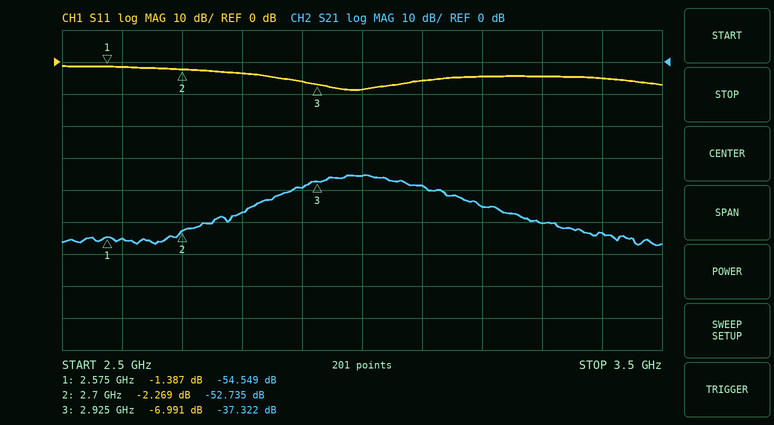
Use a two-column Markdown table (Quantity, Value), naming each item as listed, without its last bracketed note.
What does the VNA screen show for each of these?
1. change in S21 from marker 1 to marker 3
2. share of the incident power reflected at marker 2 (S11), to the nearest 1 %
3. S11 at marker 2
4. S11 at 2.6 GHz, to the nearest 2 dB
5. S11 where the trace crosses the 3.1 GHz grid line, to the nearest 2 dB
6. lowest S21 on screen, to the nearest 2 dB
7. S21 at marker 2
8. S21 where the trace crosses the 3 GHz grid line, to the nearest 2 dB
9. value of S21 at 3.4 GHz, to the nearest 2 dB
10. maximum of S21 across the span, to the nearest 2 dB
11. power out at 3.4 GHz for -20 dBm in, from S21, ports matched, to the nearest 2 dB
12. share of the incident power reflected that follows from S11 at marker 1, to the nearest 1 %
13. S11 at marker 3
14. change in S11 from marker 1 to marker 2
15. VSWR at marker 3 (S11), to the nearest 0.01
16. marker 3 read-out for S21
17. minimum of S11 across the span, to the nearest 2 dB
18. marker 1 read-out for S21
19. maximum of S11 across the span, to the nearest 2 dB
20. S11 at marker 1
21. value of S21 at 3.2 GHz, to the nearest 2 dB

| Quantity | Value |
|---|---|
| change in S21 from marker 1 to marker 3 | 17.227 dB |
| share of the incident power reflected at marker 2 (S11), to the nearest 1 % | 59 % |
| S11 at marker 2 | -2.269 dB |
| S11 at 2.6 GHz, to the nearest 2 dB | -2 dB |
| S11 where the trace crosses the 3.1 GHz grid line, to the nearest 2 dB | -6 dB |
| lowest S21 on screen, to the nearest 2 dB | -58 dB |
| S21 at marker 2 | -52.735 dB |
| S21 where the trace crosses the 3 GHz grid line, to the nearest 2 dB | -36 dB |
| value of S21 at 3.4 GHz, to the nearest 2 dB | -54 dB |
| maximum of S21 across the span, to the nearest 2 dB | -36 dB |
| power out at 3.4 GHz for -20 dBm in, from S21, ports matched, to the nearest 2 dB | -74 dBm |
| share of the incident power reflected that follows from S11 at marker 1, to the nearest 1 % | 73 % |
| S11 at marker 3 | -6.991 dB |
| change in S11 from marker 1 to marker 2 | -0.882 dB |
| VSWR at marker 3 (S11), to the nearest 0.01 | 2.62 |
| marker 3 read-out for S21 | -37.322 dB |
| minimum of S11 across the span, to the nearest 2 dB | -8 dB |
| marker 1 read-out for S21 | -54.549 dB |
| maximum of S11 across the span, to the nearest 2 dB | -2 dB |
| S11 at marker 1 | -1.387 dB |
| value of S21 at 3.2 GHz, to the nearest 2 dB | -46 dB |
